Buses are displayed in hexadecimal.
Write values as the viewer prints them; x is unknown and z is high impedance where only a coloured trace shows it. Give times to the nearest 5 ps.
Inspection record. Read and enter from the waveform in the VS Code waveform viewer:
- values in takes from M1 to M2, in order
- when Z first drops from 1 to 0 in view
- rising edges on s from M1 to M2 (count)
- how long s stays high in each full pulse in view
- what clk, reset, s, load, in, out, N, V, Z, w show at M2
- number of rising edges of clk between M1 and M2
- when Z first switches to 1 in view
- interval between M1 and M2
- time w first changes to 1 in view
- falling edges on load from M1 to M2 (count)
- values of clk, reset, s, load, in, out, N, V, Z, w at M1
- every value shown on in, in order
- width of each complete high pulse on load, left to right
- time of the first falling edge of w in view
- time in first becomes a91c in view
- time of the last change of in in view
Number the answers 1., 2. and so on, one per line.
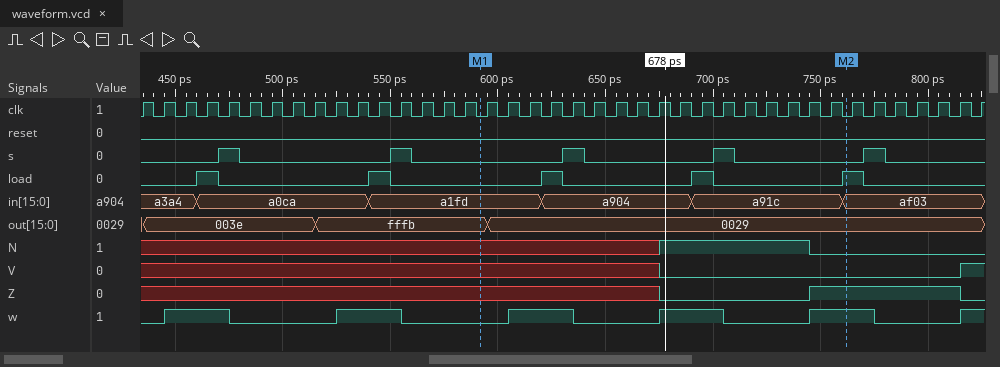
1. a1fd, a904, a91c, af03
2. 815 ps
3. 2
4. 10 ps, 10 ps, 10 ps, 10 ps, 10 ps
5. clk=0, reset=0, s=0, load=1, in=af03, out=0029, N=0, V=0, Z=1, w=1
6. 17
7. 745 ps
8. 170 ps
9. 445 ps
10. 2
11. clk=0, reset=0, s=0, load=0, in=a1fd, out=fffb, N=x, V=x, Z=x, w=0
12. a3a4, a0ca, a1fd, a904, a91c, af03
13. 10 ps, 10 ps, 10 ps, 10 ps, 10 ps
14. 475 ps
15. 690 ps
16. 760 ps
